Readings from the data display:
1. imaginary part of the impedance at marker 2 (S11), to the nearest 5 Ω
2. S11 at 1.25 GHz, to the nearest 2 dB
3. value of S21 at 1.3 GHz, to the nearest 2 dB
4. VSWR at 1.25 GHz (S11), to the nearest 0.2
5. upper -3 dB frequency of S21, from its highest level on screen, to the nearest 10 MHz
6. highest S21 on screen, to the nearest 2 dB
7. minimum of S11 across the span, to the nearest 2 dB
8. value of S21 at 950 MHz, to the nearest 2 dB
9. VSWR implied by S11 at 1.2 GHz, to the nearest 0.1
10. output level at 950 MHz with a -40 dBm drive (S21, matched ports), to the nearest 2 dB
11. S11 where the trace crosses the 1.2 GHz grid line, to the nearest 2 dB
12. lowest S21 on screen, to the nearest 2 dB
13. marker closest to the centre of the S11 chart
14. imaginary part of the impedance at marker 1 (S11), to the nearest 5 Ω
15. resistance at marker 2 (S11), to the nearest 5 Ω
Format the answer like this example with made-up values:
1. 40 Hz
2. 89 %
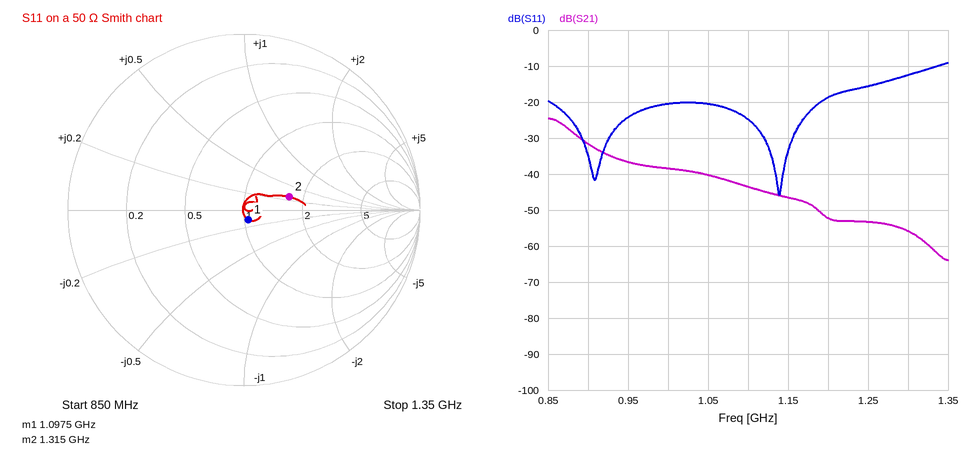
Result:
1. +15 Ω
2. -16 dB
3. -56 dB
4. 1.4
5. 880 MHz
6. -24 dB
7. -46 dB
8. -36 dB
9. 1.3
10. -76 dBm
11. -18 dB
12. -64 dB
13. marker 1
14. -5 Ω
15. 85 Ω
